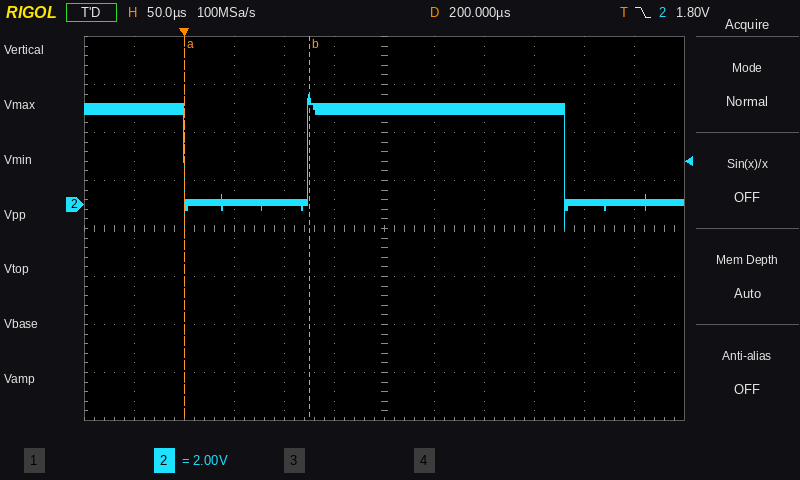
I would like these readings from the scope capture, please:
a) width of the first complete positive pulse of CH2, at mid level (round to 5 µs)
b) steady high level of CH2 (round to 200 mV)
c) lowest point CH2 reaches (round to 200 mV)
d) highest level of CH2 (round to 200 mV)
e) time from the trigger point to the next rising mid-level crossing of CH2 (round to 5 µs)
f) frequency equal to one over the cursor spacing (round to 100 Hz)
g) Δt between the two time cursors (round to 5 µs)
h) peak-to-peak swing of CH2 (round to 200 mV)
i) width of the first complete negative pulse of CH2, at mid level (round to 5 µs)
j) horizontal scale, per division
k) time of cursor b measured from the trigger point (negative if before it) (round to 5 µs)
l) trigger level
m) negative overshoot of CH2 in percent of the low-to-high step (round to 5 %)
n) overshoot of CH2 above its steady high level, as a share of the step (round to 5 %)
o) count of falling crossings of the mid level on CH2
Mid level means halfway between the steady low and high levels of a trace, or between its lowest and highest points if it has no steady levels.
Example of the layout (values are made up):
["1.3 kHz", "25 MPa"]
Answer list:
["255 µs", "4.0 V", "-1.0 V", "4.6 V", "125 µs", "8.0 kHz", "125 µs", "5.6 V", "125 µs", "50 µs", "+125 µs", "1.80 V", "30 %", "15 %", "2"]
